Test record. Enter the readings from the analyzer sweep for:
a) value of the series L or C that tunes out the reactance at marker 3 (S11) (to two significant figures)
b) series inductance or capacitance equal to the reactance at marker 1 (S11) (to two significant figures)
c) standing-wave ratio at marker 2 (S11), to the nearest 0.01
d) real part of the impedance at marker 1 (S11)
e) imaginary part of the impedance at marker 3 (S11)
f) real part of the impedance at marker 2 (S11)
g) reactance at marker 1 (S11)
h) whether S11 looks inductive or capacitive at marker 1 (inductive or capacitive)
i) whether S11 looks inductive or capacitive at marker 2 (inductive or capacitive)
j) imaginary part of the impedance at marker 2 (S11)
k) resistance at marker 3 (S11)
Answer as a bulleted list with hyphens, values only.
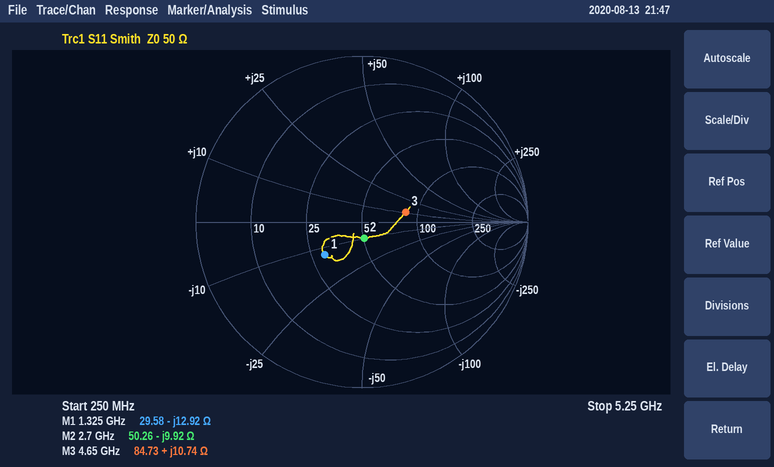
- 3.2 pF
- 9.3 pF
- 1.22
- 29.58 Ω
- +10.74 Ω
- 50.26 Ω
- -12.92 Ω
- capacitive
- capacitive
- -9.92 Ω
- 84.73 Ω
